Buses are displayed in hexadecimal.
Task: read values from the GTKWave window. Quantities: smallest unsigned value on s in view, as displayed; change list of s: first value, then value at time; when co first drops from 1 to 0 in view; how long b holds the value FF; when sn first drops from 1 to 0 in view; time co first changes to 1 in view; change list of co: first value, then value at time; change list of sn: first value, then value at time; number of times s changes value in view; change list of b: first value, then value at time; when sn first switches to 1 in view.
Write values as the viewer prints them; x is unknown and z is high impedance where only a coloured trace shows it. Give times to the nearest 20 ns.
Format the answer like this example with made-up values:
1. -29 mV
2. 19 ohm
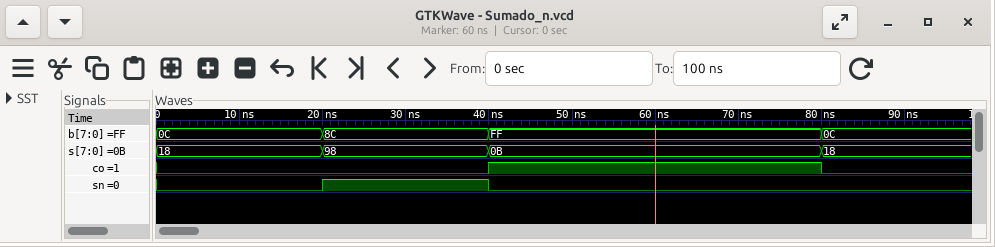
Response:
1. 0B
2. 18, 98 at 20 ns, 0B at 40 ns, 18 at 80 ns
3. 80 ns
4. 40 ns
5. 40 ns
6. 40 ns
7. 0, 1 at 40 ns, 0 at 80 ns
8. 0, 1 at 20 ns, 0 at 40 ns
9. 3
10. 0C, 8C at 20 ns, FF at 40 ns, 0C at 80 ns
11. 20 ns
